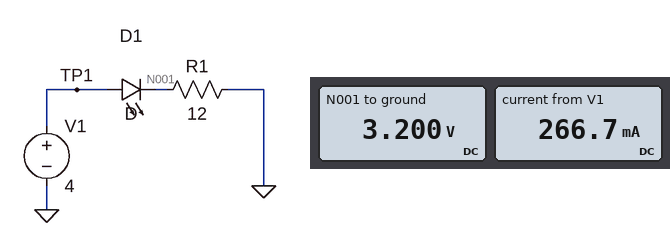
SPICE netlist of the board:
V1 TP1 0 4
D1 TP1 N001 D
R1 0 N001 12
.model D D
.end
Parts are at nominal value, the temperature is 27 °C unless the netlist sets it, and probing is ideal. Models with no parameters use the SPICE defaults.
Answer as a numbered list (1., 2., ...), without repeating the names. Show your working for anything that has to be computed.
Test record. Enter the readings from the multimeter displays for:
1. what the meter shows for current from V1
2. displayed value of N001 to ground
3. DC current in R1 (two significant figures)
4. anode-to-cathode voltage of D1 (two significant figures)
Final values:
1. 266.7 mA
2. 3.200 V
3. (3.2 V) / 12 Ω = 270 mA
4. 4 V - 3.2 V = 800 mV
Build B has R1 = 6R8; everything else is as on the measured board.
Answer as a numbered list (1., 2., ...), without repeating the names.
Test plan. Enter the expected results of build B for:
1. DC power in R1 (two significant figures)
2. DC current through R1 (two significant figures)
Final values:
1. 1.5 W
2. 470 mA
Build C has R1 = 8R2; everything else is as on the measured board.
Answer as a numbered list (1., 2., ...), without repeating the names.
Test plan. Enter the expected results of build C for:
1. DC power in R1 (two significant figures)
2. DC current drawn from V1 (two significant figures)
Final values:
1. 1.2 W
2. 390 mA
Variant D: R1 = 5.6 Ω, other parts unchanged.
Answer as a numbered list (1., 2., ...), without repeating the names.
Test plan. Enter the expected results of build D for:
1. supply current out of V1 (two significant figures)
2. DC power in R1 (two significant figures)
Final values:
1. 570 mA
2. 1.8 W
